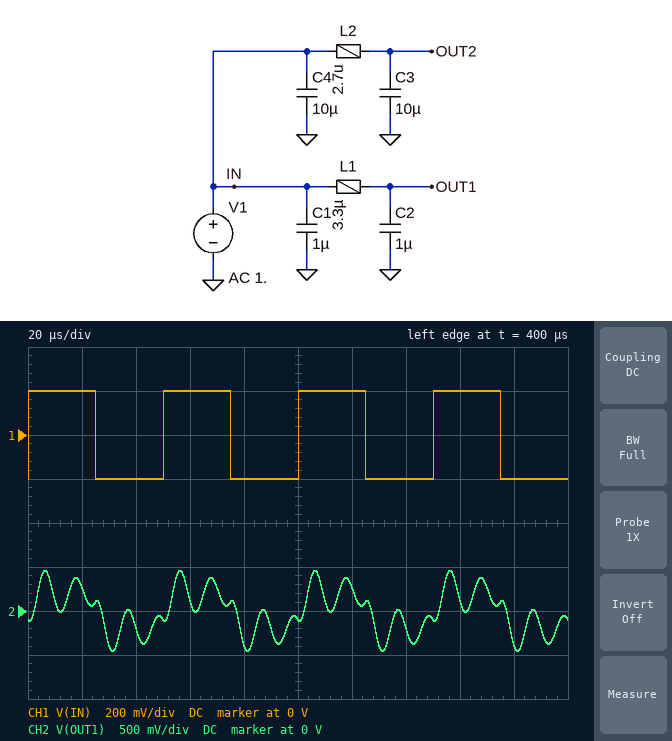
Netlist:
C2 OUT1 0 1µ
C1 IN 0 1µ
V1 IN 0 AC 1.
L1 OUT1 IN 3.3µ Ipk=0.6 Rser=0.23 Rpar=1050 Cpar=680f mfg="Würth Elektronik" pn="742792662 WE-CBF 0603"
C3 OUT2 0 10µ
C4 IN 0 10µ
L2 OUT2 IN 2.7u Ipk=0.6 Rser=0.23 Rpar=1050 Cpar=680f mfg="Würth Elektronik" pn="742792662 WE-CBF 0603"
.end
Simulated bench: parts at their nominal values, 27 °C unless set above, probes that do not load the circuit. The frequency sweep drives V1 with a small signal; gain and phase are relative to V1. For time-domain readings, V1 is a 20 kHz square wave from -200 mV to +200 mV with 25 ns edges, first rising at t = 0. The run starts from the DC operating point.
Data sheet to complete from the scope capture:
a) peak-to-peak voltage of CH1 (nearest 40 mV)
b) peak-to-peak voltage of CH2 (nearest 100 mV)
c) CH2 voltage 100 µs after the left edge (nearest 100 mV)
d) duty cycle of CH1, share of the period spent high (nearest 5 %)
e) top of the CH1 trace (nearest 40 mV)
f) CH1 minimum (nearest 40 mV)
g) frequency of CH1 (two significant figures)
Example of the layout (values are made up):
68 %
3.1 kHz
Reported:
400 mV
900 mV
-100 mV
50 %
200 mV
-200 mV
20 kHz
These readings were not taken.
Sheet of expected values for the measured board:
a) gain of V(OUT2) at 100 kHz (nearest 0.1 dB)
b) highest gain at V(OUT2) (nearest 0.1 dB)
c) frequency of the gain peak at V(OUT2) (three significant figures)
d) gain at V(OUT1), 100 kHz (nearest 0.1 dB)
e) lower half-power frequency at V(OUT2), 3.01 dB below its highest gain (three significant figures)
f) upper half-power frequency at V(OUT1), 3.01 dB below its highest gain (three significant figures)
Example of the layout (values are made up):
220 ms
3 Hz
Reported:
-19.8 dB
7.3 dB
29.1 kHz
9.5 dB
21.0 kHz
92.7 kHz
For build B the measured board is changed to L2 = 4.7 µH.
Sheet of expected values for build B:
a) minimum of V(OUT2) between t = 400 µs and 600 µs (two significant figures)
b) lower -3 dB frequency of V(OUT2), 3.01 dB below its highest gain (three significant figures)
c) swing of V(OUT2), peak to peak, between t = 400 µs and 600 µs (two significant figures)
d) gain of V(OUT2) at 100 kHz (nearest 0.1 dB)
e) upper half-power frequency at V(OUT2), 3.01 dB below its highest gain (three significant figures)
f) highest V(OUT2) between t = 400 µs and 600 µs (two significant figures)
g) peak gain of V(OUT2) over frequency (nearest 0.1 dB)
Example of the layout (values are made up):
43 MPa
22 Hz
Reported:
-650 mV
18.2 kHz
1.3 V
-24.9 dB
26.2 kHz
650 mV
9.6 dB
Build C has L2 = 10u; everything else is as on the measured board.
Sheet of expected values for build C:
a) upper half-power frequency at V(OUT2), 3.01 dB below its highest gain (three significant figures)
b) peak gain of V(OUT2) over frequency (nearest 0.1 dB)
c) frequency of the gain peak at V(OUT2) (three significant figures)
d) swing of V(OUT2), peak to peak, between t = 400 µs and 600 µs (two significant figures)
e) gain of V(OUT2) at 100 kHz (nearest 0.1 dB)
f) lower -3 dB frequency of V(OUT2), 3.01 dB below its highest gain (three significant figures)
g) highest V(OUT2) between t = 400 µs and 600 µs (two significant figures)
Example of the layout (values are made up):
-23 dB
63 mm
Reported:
17.5 kHz
12.8 dB
15.7 kHz
780 mV
-31.7 dB
13.7 kHz
390 mV
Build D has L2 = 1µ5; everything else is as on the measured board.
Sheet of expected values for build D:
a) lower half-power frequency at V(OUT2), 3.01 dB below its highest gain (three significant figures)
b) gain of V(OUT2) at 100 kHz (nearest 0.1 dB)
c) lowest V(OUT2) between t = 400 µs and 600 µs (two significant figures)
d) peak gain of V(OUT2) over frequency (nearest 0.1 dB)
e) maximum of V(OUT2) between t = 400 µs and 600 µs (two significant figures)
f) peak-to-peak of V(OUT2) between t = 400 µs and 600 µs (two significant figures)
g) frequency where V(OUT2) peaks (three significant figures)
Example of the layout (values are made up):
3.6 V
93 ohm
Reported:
20.8 kHz
-14.2 dB
-330 mV
4.9 dB
330 mV
660 mV
37.3 kHz
